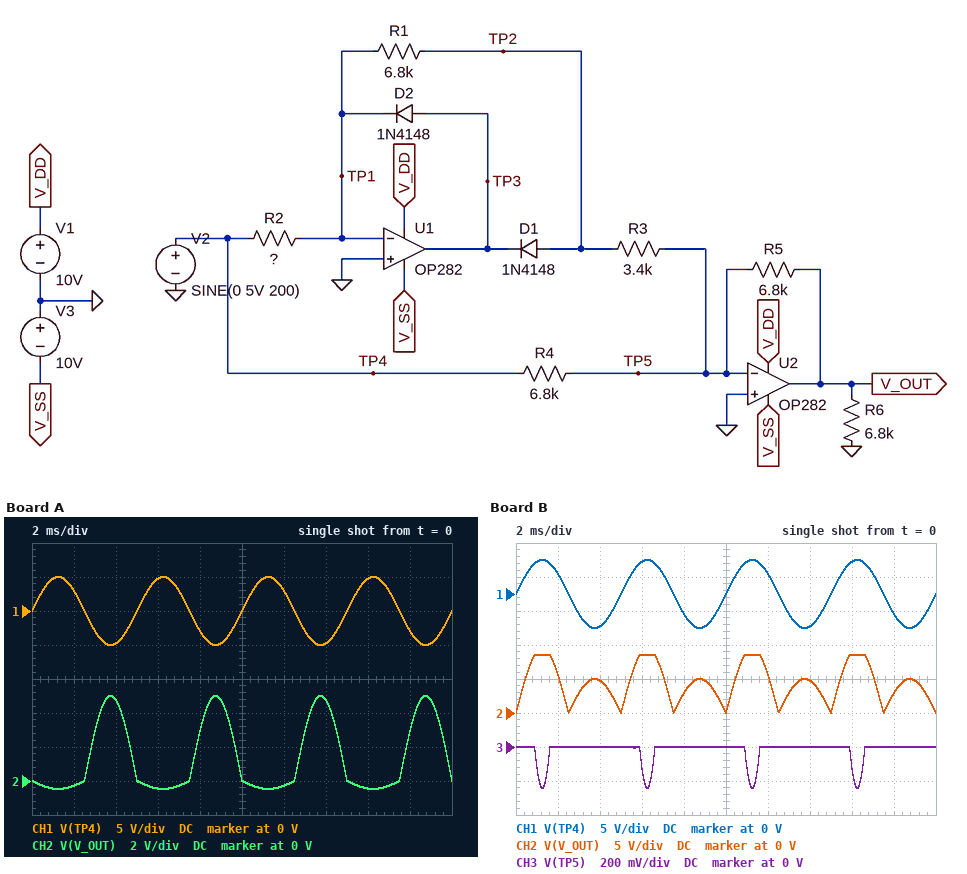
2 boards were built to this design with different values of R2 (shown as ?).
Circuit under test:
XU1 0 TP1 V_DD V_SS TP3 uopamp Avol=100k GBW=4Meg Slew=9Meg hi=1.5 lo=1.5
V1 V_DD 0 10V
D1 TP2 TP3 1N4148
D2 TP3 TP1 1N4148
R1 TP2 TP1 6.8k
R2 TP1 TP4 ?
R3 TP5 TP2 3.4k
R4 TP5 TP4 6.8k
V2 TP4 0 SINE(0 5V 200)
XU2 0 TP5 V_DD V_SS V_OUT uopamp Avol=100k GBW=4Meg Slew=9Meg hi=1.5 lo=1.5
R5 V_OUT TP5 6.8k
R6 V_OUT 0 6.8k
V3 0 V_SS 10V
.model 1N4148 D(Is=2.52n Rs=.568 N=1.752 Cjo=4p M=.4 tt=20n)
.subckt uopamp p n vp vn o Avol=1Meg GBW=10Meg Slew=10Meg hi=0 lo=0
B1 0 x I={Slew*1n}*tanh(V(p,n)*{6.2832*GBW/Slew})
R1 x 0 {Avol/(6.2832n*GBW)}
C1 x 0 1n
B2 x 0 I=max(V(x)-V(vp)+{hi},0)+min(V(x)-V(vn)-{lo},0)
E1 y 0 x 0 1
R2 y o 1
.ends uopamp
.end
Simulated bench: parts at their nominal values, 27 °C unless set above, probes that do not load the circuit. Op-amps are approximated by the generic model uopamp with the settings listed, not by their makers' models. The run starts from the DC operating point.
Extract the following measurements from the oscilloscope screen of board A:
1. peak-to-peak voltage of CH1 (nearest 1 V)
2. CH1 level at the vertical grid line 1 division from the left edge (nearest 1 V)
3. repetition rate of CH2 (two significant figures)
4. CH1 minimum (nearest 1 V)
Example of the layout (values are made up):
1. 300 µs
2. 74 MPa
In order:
1. 10 V
2. 3 V
3. 200 Hz
4. -5 V
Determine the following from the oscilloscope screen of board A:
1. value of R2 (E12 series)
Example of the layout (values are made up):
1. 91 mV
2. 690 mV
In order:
1. 15 kΩ
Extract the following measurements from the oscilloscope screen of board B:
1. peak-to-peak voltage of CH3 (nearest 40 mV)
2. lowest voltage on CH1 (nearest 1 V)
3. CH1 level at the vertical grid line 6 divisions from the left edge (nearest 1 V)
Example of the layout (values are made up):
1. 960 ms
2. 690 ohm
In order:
1. 240 mV
2. -5 V
3. 3 V
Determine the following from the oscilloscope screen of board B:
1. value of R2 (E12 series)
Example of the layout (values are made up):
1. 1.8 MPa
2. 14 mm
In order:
1. 4.7 kΩ
